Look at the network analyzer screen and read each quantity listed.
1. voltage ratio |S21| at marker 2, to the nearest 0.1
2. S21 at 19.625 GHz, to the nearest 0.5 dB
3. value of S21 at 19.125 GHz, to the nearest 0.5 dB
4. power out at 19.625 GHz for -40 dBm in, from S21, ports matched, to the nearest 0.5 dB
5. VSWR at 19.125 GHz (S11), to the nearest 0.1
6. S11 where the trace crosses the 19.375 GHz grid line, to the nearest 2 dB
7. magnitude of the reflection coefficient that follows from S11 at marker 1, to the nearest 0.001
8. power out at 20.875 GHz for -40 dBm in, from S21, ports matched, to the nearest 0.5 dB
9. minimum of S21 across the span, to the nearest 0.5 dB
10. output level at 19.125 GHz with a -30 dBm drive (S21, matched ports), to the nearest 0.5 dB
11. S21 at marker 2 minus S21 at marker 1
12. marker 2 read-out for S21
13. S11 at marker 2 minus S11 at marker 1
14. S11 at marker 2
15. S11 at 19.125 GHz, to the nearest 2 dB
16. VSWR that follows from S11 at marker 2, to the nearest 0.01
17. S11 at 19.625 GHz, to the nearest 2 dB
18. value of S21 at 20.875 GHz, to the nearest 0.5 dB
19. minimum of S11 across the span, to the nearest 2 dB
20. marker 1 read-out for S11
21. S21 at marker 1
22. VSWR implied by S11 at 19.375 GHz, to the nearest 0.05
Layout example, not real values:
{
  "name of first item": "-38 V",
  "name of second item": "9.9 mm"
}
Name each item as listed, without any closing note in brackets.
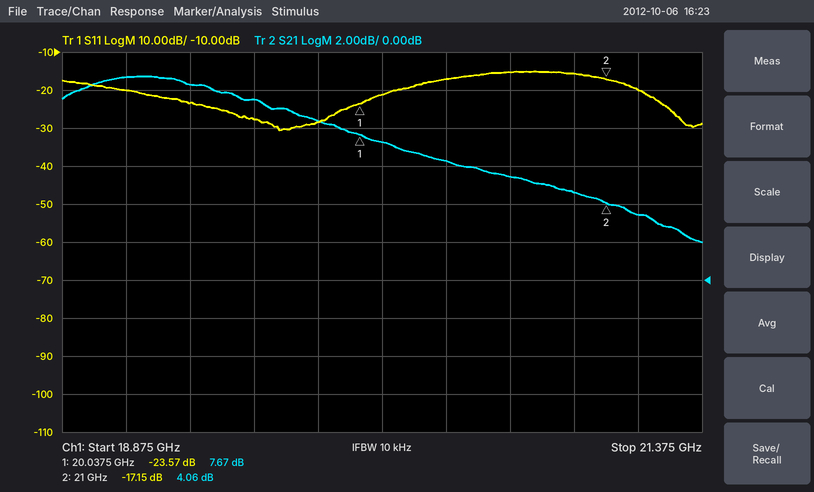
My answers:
{
  "voltage ratio |S21| at marker 2, to the nearest 0.1": "1.6",
  "S21 at 19.625 GHz, to the nearest 0.5 dB": "9.5 dB",
  "value of S21 at 19.125 GHz, to the nearest 0.5 dB": "10.5 dB",
  "power out at 19.625 GHz for -40 dBm in, from S21, ports matched, to the nearest 0.5 dB": "-30.5 dBm",
  "VSWR at 19.125 GHz (S11), to the nearest 0.1": "1.2",
  "S11 where the trace crosses the 19.375 GHz grid line, to the nearest 2 dB": "-24 dB",
  "magnitude of the reflection coefficient that follows from S11 at marker 1, to the nearest 0.001": "0.066",
  "power out at 20.875 GHz for -40 dBm in, from S21, ports matched, to the nearest 0.5 dB": "-35.5 dBm",
  "minimum of S21 across the span, to the nearest 0.5 dB": "2.0 dB",
  "output level at 19.125 GHz with a -30 dBm drive (S21, matched ports), to the nearest 0.5 dB": "-19.5 dBm",
  "S21 at marker 2 minus S21 at marker 1": "-3.61 dB",
  "marker 2 read-out for S21": "4.06 dB",
  "S11 at marker 2 minus S11 at marker 1": "6.42 dB",
  "S11 at marker 2": "-17.15 dB",
  "S11 at 19.125 GHz, to the nearest 2 dB": "-20 dB",
  "VSWR that follows from S11 at marker 2, to the nearest 0.01": "1.32",
  "S11 at 19.625 GHz, to the nearest 2 dB": "-28 dB",
  "value of S21 at 20.875 GHz, to the nearest 0.5 dB": "4.5 dB",
  "minimum of S11 across the span, to the nearest 2 dB": "-30 dB",
  "marker 1 read-out for S11": "-23.57 dB",
  "S21 at marker 1": "7.67 dB",
  "VSWR implied by S11 at 19.375 GHz, to the nearest 0.05": "1.15"
}
